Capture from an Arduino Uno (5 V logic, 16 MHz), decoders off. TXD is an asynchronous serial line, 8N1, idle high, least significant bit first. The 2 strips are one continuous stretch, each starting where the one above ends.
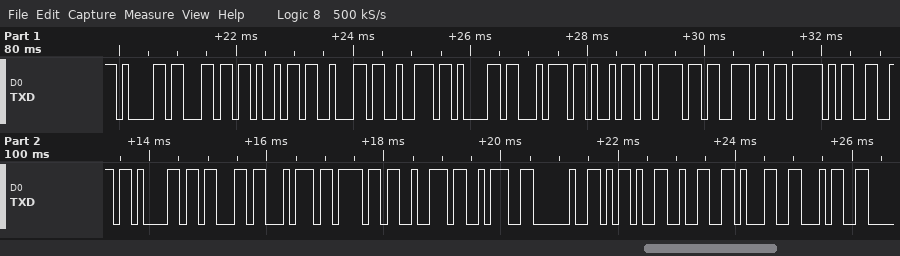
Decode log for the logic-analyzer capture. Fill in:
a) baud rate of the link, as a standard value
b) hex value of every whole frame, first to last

9600 baud
61 6C 69 62 72 61 74 69 6F 6E 5F 66 61 63 74 6F 72 3A 20 2D 32 31 34
